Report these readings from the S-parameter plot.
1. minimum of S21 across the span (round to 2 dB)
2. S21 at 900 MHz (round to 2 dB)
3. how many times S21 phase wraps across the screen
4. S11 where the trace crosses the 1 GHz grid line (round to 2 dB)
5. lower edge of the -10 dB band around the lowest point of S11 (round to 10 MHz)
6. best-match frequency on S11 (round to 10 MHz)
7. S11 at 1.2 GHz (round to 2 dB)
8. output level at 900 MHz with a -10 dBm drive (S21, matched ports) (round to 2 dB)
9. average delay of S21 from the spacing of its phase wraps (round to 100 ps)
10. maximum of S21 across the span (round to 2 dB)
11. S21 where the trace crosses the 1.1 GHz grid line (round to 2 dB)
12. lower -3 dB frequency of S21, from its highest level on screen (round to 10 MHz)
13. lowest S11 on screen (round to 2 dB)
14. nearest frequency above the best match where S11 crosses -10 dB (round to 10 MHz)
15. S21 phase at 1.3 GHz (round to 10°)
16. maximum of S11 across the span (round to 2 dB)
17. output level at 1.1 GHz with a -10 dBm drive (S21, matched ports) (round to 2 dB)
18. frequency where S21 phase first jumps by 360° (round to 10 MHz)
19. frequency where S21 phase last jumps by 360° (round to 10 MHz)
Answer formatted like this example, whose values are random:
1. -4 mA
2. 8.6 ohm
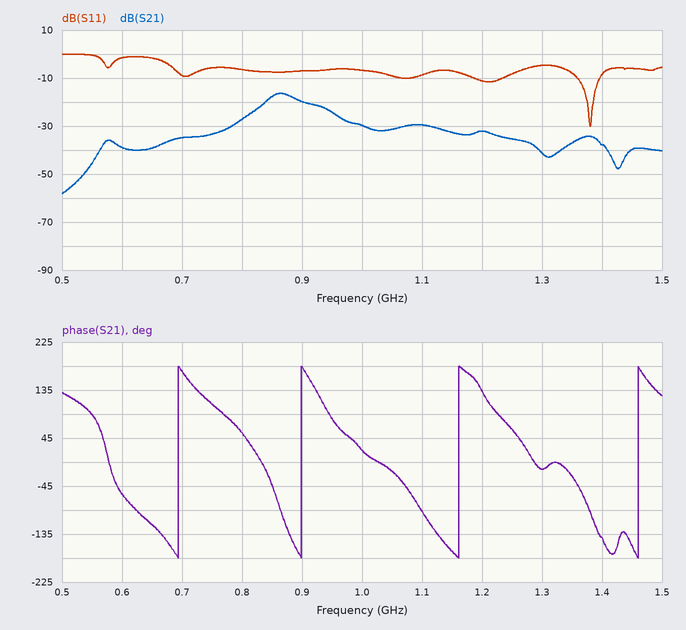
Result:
1. -58 dB
2. -20 dB
3. 4
4. -6 dB
5. 1.36 GHz
6. 1.38 GHz
7. -12 dB
8. -30 dBm
9. 3.9 ns
10. -16 dB
11. -30 dB
12. 840 MHz
13. -30 dB
14. 1.40 GHz
15. -10°
16. 0 dB
17. -40 dBm
18. 690 MHz
19. 1.46 GHz
